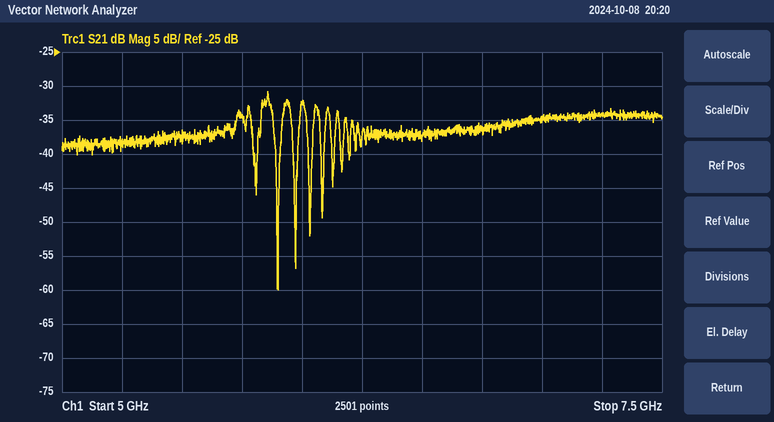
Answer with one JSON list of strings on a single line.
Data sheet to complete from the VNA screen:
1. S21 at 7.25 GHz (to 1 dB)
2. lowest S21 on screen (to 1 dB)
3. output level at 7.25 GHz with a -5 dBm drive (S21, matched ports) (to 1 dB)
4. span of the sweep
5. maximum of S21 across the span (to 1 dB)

["-34 dB", "-60 dB", "-39 dBm", "2.5 GHz", "-31 dB"]
